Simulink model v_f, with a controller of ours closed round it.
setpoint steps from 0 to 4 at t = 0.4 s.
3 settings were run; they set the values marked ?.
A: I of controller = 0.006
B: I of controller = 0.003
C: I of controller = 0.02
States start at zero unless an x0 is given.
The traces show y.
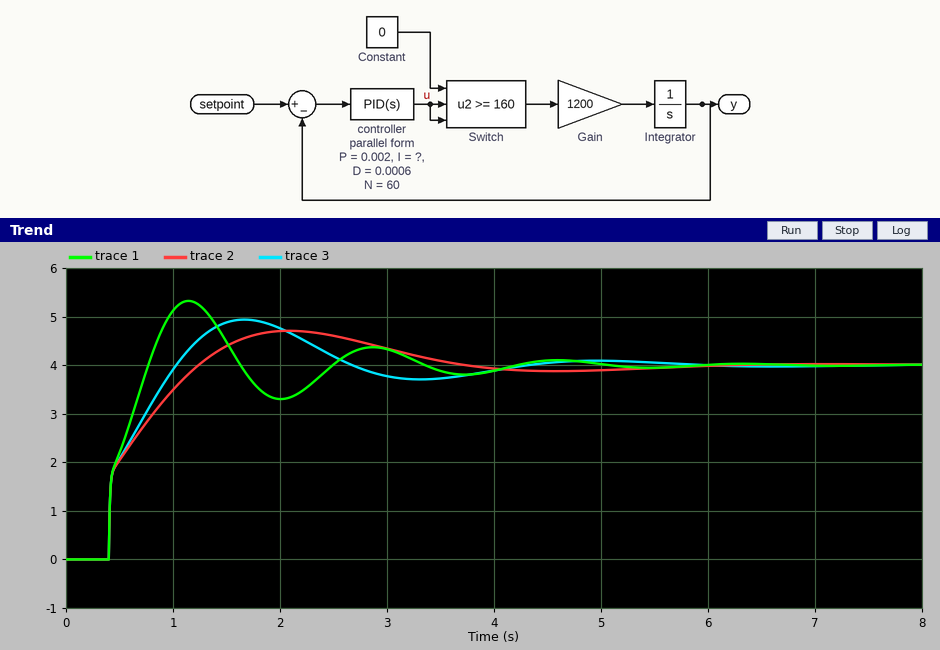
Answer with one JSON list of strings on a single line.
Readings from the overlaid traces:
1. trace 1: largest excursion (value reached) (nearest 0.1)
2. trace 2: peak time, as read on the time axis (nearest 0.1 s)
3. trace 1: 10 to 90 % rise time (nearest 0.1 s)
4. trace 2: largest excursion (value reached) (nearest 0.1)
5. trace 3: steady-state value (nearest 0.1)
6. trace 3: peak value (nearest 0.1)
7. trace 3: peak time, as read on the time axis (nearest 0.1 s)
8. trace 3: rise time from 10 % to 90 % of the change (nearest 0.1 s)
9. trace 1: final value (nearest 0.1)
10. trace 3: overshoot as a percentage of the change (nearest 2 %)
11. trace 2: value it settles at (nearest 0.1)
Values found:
["5.3", "2.1 s", "0.3 s", "4.7", "4.0", "4.9", "1.7 s", "0.5 s", "4.0", "24 %", "4.0"]
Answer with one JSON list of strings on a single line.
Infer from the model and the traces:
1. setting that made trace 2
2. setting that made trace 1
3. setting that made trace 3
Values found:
["B", "C", "A"]
